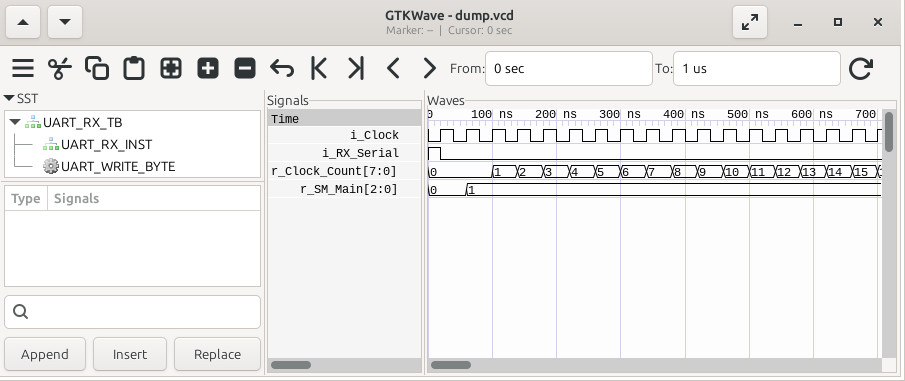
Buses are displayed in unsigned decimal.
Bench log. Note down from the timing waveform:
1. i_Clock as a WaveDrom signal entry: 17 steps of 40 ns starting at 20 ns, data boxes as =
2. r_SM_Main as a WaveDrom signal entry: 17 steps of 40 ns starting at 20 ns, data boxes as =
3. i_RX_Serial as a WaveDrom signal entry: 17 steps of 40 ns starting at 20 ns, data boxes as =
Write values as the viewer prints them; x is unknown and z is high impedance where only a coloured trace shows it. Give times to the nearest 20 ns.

{name: 'i_Clock', wave: 'p................'}
{name: 'r_SM_Main', wave: '==...............', data: '0 1'}
{name: 'i_RX_Serial', wave: '0................'}
